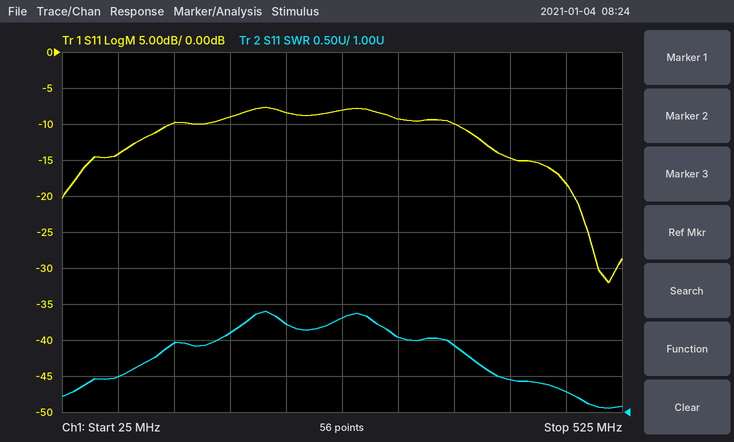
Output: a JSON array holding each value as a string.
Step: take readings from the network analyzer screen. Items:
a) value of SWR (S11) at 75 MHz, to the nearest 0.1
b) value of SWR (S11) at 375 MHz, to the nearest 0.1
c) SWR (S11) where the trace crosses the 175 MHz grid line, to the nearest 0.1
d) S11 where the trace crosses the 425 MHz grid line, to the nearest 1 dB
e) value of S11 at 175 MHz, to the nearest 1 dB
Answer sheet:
["1.5", "1.9", "2.1", "-15 dB", "-9 dB"]
